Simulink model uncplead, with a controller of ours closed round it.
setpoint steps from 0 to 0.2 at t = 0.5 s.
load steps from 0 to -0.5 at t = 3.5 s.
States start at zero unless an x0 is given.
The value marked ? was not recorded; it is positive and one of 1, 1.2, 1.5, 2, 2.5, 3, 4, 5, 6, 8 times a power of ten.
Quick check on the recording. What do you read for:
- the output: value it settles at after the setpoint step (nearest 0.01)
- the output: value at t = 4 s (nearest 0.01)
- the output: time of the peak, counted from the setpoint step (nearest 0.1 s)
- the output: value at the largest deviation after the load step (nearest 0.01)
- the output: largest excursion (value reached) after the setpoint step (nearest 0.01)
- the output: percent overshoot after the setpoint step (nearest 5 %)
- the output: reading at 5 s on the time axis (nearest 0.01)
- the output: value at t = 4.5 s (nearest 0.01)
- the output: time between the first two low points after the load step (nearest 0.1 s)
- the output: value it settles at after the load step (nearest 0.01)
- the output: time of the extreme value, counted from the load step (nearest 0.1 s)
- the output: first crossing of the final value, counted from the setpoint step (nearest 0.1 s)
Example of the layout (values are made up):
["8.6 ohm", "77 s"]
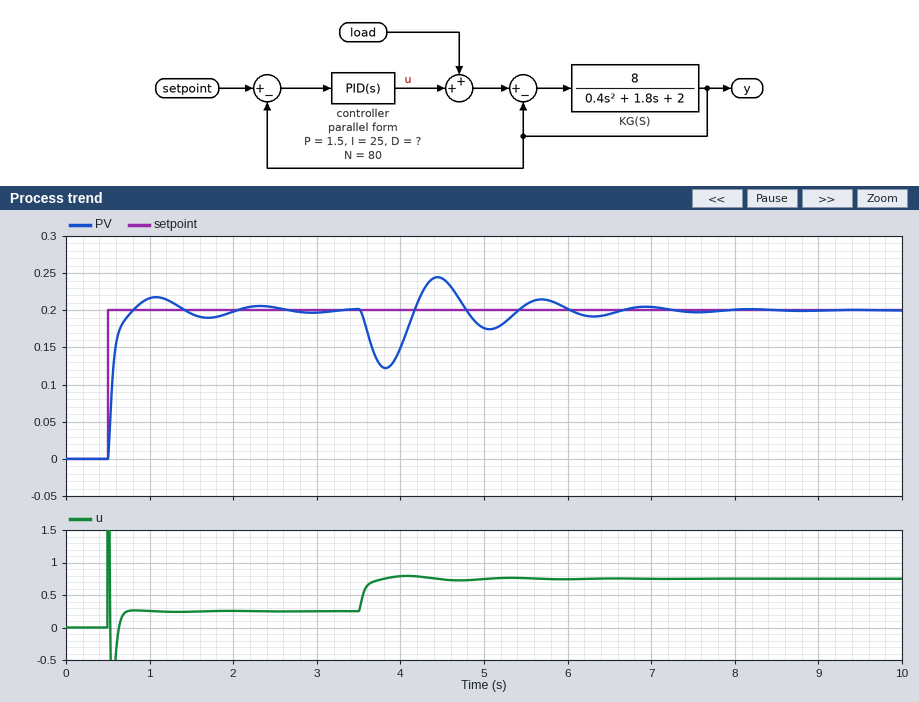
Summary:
["0.20", "0.15", "0.6 s", "0.12", "0.22", "10 %", "0.18", "0.24", "1.2 s", "0.20", "0.3 s", "0.3 s"]
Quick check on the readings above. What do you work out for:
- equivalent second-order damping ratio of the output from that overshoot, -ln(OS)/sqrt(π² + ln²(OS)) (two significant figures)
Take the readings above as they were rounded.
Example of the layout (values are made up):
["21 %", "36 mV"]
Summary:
["0.59"]
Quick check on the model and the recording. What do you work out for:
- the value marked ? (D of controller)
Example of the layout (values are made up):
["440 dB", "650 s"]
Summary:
["0.8"]
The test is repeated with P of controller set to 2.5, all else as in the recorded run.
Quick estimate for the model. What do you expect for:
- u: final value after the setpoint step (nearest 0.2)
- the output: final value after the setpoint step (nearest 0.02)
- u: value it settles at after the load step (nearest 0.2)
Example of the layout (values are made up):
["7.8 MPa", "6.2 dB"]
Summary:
["0.2", "0.20", "0.8"]
